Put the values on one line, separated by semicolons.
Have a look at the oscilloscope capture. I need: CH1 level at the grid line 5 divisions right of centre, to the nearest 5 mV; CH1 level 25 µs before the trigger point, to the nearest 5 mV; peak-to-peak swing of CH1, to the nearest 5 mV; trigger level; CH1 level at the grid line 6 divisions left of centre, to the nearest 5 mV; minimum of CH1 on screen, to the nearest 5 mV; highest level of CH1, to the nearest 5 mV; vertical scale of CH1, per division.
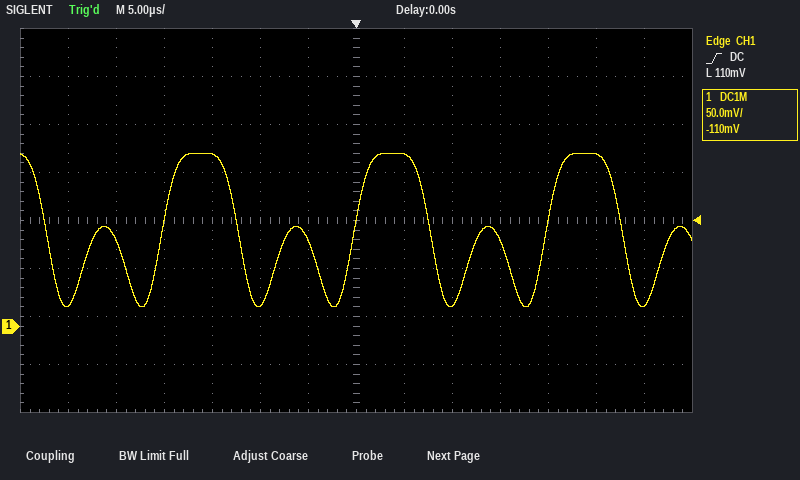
180 mV; 90 mV; 160 mV; 110 mV; 20 mV; 20 mV; 180 mV; 50 mV
